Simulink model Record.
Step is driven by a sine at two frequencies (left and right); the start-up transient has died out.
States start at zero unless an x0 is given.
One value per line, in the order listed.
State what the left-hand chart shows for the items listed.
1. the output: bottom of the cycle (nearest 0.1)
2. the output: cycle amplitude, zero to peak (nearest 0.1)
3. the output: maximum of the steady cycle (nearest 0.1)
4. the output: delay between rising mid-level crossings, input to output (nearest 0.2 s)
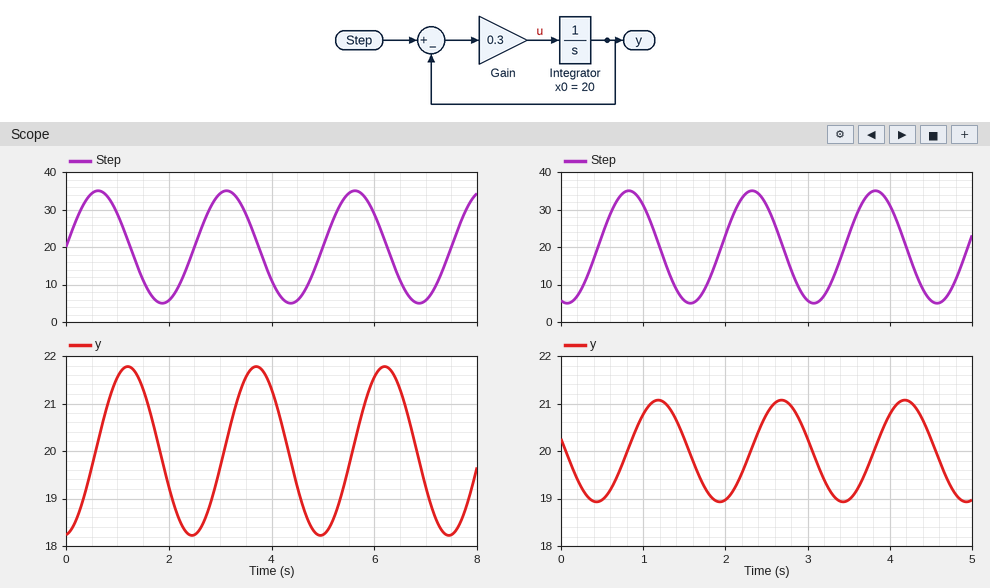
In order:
18.2
1.8
21.8
0.6 s
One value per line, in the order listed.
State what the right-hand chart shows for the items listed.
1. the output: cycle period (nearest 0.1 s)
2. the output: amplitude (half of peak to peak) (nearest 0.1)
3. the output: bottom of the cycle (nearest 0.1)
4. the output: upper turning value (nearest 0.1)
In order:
1.5 s
1.1
18.9
21.1
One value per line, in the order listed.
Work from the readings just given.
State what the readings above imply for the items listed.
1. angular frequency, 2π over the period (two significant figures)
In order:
4.2 rad/s
